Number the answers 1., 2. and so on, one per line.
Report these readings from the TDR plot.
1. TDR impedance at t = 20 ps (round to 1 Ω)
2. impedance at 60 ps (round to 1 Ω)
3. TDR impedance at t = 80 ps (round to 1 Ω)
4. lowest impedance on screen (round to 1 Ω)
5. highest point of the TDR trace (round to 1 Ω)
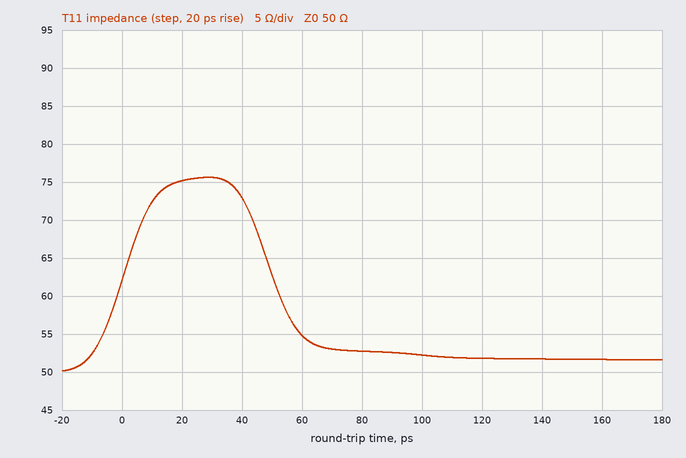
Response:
1. 75 Ω
2. 55 Ω
3. 53 Ω
4. 50 Ω
5. 76 Ω
